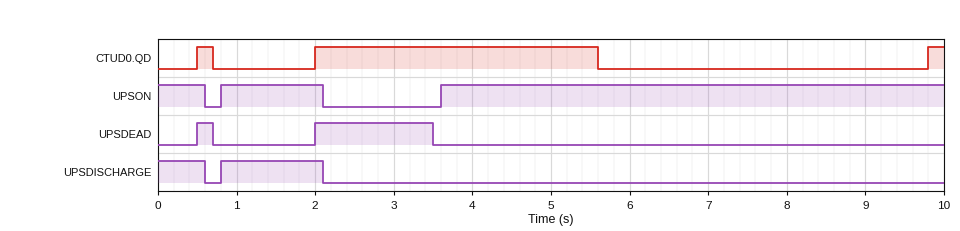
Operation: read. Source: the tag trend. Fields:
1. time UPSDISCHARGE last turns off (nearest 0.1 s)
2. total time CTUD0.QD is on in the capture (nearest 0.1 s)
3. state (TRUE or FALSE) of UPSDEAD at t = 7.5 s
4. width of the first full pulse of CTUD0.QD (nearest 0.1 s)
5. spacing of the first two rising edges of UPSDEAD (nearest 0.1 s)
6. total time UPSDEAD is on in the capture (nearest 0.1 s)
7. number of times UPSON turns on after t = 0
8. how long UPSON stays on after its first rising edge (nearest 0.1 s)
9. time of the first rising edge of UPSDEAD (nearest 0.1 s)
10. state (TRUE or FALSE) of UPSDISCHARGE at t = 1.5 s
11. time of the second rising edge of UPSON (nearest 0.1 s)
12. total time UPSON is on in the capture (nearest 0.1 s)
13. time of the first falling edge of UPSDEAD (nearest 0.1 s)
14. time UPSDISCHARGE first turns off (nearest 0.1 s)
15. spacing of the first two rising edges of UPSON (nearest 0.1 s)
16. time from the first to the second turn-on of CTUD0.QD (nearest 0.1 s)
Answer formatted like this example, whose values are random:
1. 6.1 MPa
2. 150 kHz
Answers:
1. 2.1 s
2. 4.0 s
3. FALSE
4. 0.2 s
5. 1.5 s
6. 1.7 s
7. 2
8. 1.3 s
9. 0.5 s
10. TRUE
11. 3.6 s
12. 8.3 s
13. 0.7 s
14. 0.6 s
15. 2.8 s
16. 1.5 s
